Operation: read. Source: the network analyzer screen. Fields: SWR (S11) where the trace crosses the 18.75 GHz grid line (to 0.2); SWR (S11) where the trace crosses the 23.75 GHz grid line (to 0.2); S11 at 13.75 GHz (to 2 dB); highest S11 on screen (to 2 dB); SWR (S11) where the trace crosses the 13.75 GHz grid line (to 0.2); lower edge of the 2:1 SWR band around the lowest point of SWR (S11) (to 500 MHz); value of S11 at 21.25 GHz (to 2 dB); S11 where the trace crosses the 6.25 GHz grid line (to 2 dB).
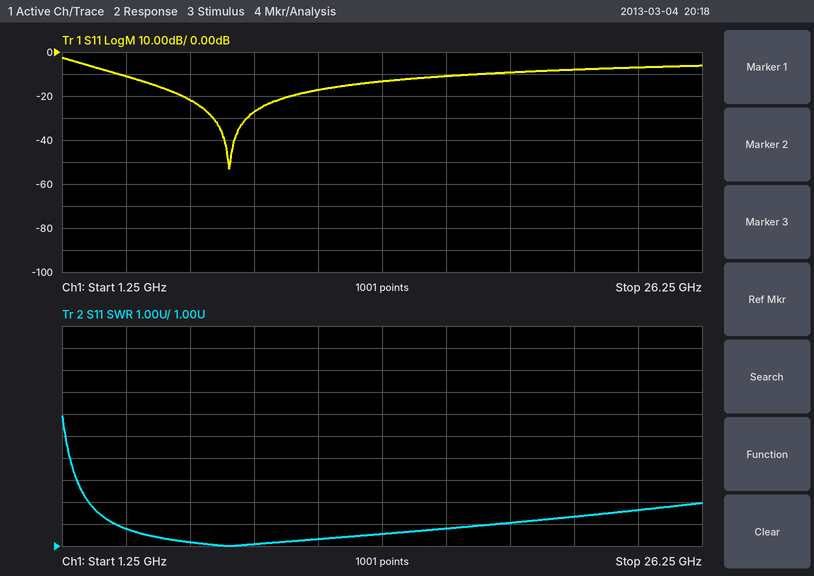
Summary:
2.0
2.6
-14 dB
-2 dB
1.6
3.5 GHz
-8 dB
-22 dB
